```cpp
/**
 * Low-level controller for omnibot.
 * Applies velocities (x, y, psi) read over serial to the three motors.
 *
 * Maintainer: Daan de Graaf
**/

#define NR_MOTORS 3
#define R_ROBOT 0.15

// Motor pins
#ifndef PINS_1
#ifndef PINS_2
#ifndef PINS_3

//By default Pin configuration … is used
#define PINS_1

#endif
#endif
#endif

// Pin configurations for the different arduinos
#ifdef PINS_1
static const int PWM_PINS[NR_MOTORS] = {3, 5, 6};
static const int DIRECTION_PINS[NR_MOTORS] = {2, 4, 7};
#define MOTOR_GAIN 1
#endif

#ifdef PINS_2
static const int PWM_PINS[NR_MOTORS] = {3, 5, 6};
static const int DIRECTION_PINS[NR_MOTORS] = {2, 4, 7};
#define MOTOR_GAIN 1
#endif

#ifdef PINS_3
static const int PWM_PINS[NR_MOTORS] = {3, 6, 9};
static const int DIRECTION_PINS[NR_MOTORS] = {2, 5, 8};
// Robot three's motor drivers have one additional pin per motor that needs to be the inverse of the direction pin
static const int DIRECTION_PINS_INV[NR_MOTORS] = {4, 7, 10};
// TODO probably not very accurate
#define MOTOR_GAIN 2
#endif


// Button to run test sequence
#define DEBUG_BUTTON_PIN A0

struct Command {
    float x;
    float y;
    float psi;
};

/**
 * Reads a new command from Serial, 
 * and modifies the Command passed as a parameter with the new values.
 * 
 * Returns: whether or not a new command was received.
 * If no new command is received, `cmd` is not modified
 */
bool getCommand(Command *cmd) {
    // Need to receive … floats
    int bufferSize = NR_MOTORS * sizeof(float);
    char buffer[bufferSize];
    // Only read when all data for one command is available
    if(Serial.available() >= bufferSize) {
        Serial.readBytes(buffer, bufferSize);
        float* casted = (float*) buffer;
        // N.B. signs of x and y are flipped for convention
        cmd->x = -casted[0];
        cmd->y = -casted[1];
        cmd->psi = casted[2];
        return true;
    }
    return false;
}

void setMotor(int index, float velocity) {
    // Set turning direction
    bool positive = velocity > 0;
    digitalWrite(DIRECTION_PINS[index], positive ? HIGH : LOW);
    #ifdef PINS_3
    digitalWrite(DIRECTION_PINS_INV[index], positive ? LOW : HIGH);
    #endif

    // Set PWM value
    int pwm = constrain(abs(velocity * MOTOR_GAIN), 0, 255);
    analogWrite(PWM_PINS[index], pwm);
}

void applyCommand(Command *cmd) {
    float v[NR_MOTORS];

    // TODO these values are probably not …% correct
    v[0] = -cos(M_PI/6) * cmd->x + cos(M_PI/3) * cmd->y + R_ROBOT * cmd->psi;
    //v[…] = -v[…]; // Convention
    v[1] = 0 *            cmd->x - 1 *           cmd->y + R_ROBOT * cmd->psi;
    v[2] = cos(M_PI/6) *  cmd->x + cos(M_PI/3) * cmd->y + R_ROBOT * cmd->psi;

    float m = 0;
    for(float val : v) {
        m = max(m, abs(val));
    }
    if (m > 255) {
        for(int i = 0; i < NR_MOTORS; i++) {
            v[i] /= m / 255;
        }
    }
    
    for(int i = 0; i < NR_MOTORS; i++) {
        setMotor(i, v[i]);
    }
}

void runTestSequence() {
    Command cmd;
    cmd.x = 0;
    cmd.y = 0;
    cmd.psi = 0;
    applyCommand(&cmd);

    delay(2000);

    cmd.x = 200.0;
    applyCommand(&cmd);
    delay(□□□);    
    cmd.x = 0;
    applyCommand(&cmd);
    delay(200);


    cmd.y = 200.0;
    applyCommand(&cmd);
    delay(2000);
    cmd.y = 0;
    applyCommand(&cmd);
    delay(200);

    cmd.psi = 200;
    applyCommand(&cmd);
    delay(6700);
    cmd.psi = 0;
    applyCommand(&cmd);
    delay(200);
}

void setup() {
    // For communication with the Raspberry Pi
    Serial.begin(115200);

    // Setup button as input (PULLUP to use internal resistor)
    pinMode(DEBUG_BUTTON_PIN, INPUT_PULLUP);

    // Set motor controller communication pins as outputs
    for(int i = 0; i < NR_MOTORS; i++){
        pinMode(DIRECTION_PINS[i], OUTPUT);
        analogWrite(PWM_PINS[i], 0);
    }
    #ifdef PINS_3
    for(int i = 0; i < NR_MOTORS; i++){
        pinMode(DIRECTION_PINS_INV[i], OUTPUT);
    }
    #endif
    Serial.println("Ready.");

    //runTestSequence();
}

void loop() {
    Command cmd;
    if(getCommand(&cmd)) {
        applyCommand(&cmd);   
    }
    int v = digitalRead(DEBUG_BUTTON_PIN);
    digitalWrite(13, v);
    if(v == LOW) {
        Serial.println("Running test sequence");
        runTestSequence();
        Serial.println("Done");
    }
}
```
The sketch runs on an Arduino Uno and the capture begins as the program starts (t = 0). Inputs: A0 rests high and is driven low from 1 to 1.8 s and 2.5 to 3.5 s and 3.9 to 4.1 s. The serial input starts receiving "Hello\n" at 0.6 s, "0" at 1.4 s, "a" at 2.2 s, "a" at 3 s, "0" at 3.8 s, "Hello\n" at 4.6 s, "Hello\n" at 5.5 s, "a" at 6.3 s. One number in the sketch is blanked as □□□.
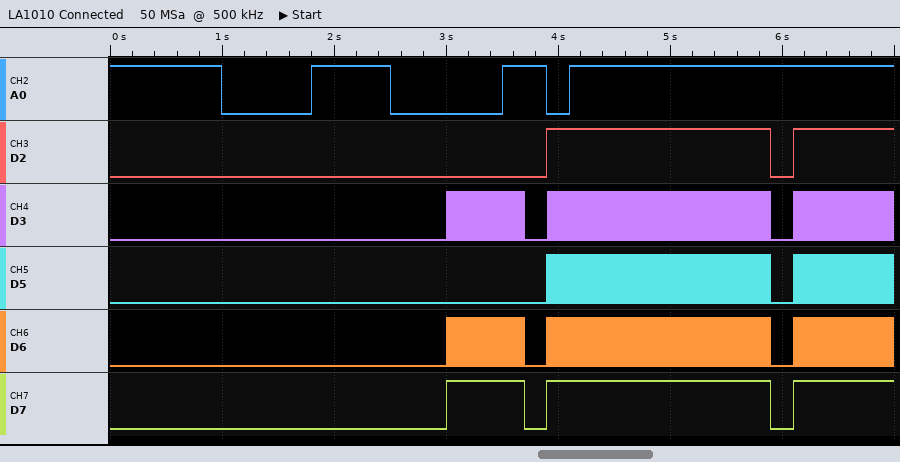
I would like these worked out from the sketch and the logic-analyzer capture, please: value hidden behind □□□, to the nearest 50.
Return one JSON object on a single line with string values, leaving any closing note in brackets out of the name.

{"value hidden behind □□□, to the nearest 50": "700"}
